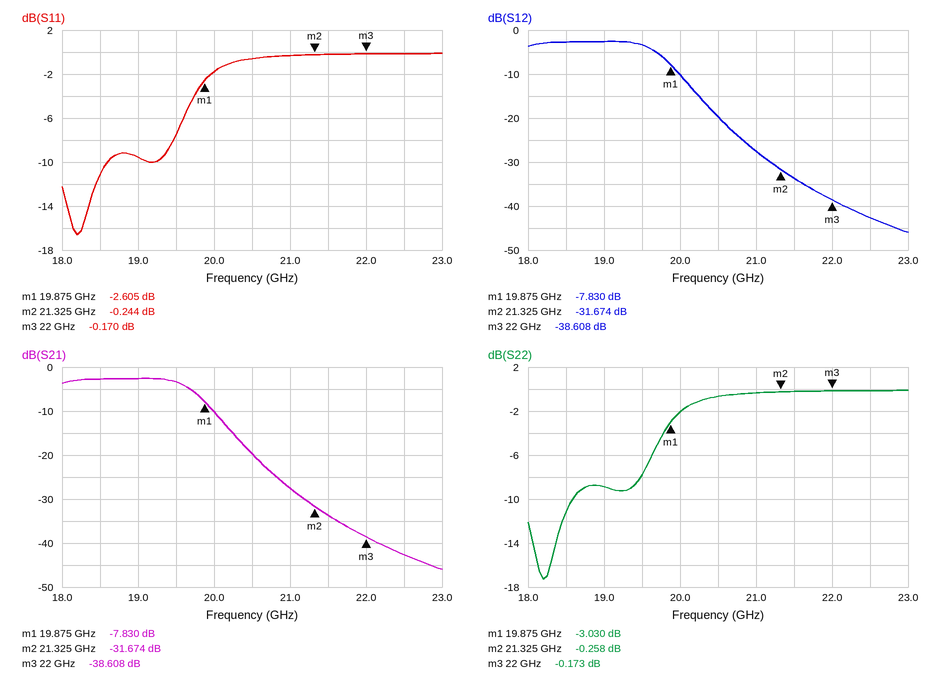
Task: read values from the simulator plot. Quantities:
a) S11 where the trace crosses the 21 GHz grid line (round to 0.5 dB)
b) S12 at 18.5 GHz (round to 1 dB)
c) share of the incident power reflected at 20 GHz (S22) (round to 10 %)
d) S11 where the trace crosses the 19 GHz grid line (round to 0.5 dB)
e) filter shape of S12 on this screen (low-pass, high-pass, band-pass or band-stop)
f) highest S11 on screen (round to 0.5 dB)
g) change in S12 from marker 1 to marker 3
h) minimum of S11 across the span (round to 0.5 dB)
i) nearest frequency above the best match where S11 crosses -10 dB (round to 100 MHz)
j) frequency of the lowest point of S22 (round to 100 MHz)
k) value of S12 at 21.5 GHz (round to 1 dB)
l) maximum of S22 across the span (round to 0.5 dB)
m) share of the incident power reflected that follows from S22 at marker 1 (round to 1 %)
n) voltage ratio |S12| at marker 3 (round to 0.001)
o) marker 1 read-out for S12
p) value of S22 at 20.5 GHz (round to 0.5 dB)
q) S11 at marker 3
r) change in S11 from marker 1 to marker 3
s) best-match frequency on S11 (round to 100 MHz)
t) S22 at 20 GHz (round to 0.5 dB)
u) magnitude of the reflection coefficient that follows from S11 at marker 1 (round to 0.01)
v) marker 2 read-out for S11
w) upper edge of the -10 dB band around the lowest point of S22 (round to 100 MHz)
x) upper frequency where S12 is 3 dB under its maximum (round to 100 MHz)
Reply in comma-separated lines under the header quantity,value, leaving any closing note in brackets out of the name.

quantity,value
S11 where the trace crosses the 21 GHz grid line,-0.5 dB
S12 at 18.5 GHz,-3 dB
share of the incident power reflected at 20 GHz (S22),60 %
S11 where the trace crosses the 19 GHz grid line,-9.5 dB
filter shape of S12 on this screen,low-pass
highest S11 on screen,0.0 dB
change in S12 from marker 1 to marker 3,-30.778 dB
minimum of S11 across the span,-16.5 dB
nearest frequency above the best match where S11 crosses -10 dB,18.6 GHz
frequency of the lowest point of S22,18.2 GHz
value of S12 at 21.5 GHz,-34 dB
maximum of S22 across the span,0.0 dB
share of the incident power reflected that follows from S22 at marker 1,50 %
voltage ratio |S12| at marker 3,0.012
marker 1 read-out for S12,-7.830 dB
value of S22 at 20.5 GHz,-0.5 dB
S11 at marker 3,-0.170 dB
change in S11 from marker 1 to marker 3,2.435 dB
best-match frequency on S11,18.2 GHz
S22 at 20 GHz,-2.0 dB
magnitude of the reflection coefficient that follows from S11 at marker 1,0.74
marker 2 read-out for S11,-0.244 dB
upper edge of the -10 dB band around the lowest point of S22,18.6 GHz
upper frequency where S12 is 3 dB under its maximum,19.7 GHz
